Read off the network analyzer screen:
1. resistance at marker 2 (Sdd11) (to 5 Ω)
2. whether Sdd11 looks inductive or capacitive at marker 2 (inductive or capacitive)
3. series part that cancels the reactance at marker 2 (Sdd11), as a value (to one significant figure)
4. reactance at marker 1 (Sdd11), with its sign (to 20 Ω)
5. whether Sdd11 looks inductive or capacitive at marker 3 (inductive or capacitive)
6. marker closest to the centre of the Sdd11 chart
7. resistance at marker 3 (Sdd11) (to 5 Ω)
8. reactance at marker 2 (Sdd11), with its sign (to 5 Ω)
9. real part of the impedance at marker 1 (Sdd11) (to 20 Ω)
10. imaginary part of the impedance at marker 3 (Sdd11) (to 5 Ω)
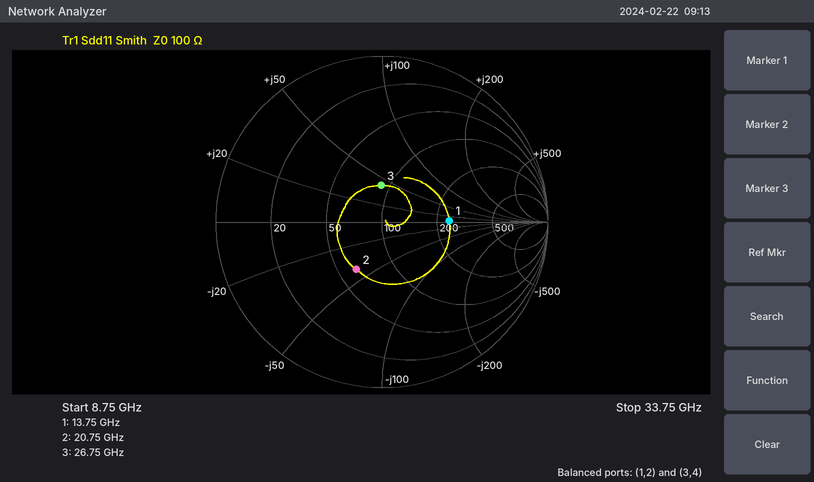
65 Ω
capacitive
300 pH
0 Ω
inductive
marker 3
90 Ω
-40 Ω
240 Ω
+40 Ω
